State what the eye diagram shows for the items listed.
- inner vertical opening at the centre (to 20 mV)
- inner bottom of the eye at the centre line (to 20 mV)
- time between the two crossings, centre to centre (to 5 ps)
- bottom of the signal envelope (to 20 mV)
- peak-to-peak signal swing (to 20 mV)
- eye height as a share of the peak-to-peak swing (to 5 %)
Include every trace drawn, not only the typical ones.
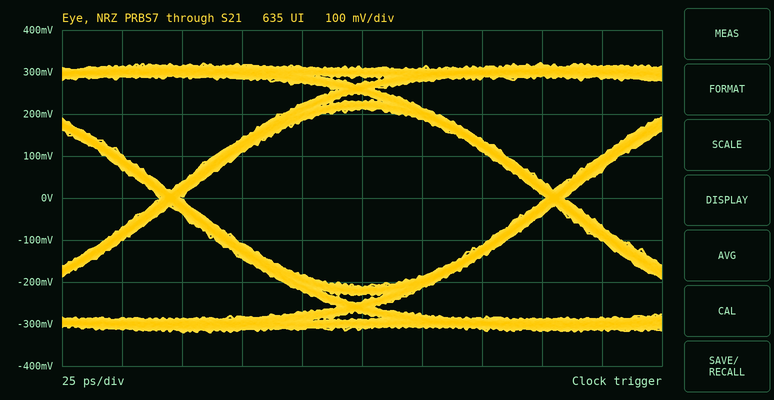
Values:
420 mV
-220 mV
160 ps
-320 mV
640 mV
65 %
